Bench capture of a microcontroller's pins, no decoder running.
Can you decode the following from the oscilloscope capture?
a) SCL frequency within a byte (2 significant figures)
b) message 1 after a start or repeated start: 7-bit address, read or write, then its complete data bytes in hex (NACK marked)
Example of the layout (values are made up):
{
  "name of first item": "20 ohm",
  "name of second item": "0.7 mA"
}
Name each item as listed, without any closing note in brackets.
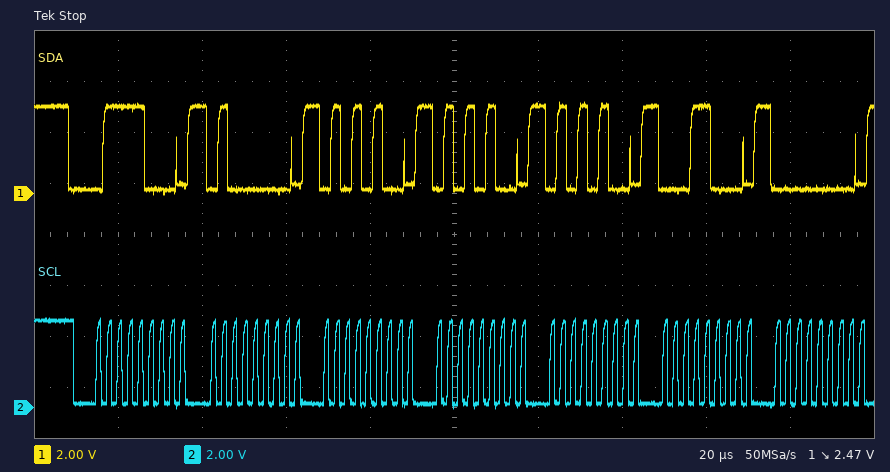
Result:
{
  "SCL frequency within a byte": "400 kHz",
  "message 1 after a start or repeated start: 7-bit address, read or write, then its complete data bytes in hex": "0x3C write: 40 54 54 54 18 00"
}
